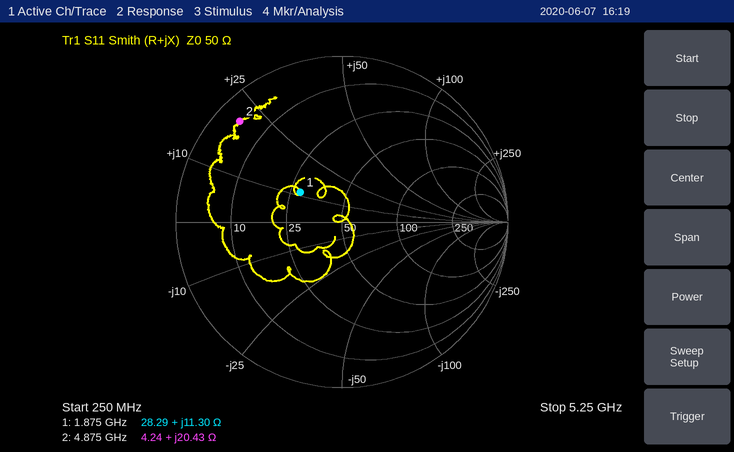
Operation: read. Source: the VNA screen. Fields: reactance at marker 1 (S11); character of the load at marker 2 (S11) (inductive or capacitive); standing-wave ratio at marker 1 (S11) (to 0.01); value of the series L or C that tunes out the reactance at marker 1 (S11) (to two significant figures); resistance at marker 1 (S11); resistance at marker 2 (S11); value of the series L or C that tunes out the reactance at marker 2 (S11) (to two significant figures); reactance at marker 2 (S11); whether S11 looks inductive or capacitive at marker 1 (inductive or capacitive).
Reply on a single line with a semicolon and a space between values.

+11.30 Ω; inductive; 1.90; 7.5 pF; 28.29 Ω; 4.24 Ω; 1.6 pF; +20.43 Ω; inductive
